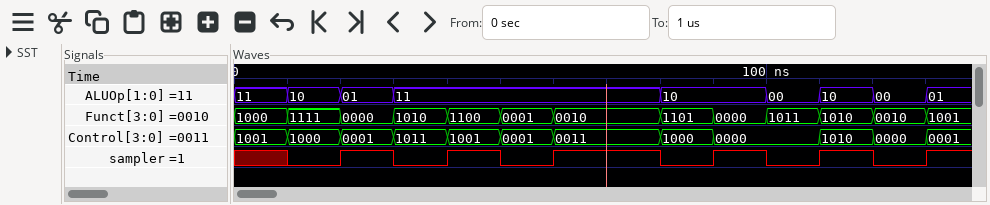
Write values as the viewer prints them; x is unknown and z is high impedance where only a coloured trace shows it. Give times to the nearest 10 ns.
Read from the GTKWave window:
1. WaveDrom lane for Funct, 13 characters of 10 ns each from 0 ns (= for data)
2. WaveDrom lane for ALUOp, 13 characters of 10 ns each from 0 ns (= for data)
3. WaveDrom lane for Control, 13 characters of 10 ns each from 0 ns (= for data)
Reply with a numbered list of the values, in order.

1. {name: 'Funct', wave: '=======.=====', data: '1000 1111 0000 1010 1100 0001 0010 1101 0000 1011 1010 0010'}
2. {name: 'ALUOp', wave: '====....=.===', data: '11 10 01 11 10 00 10 00'}
3. {name: 'Control', wave: '=======.==.==', data: '1001 1000 0001 1011 1001 0001 0011 1000 0000 1010 0000'}
